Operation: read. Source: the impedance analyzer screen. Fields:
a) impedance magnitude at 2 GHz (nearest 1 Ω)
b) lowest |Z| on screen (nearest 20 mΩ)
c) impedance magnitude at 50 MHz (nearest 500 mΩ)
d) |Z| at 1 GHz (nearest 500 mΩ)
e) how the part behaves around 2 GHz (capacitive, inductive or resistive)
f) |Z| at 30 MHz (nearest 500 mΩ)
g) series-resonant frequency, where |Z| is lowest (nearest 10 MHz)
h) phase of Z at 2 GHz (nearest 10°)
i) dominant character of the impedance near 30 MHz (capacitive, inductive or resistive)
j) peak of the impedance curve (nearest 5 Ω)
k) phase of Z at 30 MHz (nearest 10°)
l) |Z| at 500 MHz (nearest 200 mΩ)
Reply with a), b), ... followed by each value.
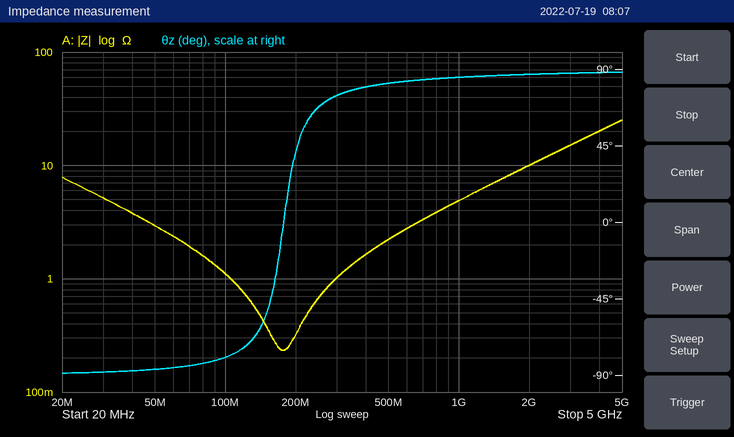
a) 10 Ω
b) 240 mΩ
c) 3.0 Ω
d) 5.0 Ω
e) inductive
f) 5.0 Ω
g) 180 MHz
h) 90°
i) capacitive
j) 25 Ω
k) -90°
l) 2.2 Ω
